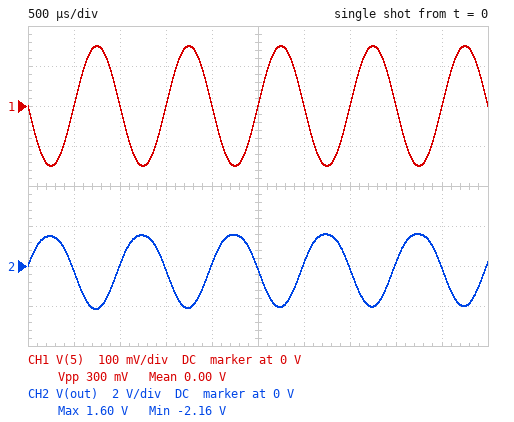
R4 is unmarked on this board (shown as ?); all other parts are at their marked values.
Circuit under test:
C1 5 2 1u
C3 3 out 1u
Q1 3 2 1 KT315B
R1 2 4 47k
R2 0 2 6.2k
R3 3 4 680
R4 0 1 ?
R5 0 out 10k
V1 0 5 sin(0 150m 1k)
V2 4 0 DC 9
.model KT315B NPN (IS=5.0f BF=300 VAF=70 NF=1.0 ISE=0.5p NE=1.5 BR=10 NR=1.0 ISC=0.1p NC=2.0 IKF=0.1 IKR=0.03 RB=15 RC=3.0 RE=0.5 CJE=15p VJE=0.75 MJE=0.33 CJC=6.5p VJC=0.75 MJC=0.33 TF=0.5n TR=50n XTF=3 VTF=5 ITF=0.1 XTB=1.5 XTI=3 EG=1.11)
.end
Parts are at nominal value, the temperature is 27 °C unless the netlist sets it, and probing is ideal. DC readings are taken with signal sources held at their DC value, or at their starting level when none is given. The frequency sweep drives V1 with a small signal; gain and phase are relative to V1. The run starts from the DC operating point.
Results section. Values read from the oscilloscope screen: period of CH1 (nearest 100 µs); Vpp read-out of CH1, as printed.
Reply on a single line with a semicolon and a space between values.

1.0 ms; 300 mV
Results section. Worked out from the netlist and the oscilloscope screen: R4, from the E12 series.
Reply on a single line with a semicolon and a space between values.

39 Ω
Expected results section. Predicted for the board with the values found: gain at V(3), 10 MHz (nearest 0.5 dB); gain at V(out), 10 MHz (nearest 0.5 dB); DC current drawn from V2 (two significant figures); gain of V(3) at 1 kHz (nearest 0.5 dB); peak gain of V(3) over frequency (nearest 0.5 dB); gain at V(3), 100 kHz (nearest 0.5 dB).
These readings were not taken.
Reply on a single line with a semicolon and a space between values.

22.0 dB; 22.0 dB; 3.1 mA; 22.0 dB; 22.0 dB; 22.0 dB
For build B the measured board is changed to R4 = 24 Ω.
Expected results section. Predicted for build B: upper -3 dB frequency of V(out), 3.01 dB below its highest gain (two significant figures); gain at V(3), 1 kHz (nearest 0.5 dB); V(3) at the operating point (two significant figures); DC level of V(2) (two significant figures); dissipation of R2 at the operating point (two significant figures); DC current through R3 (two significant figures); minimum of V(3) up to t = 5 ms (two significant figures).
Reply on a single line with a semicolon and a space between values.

48 MHz; 25.5 dB; 6.7 V; 790 mV; 100 µW; 3.4 mA; 3.4 V
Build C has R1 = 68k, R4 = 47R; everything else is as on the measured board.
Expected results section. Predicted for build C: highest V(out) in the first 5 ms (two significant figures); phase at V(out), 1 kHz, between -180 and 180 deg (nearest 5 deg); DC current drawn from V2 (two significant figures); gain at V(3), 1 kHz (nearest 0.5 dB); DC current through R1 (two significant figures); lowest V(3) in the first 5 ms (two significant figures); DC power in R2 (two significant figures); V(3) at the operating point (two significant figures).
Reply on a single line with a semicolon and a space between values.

430 mV; 5 deg; 670 µA; 16.5 dB; 120 µA; 7.2 V; 75 µW; 8.6 V
